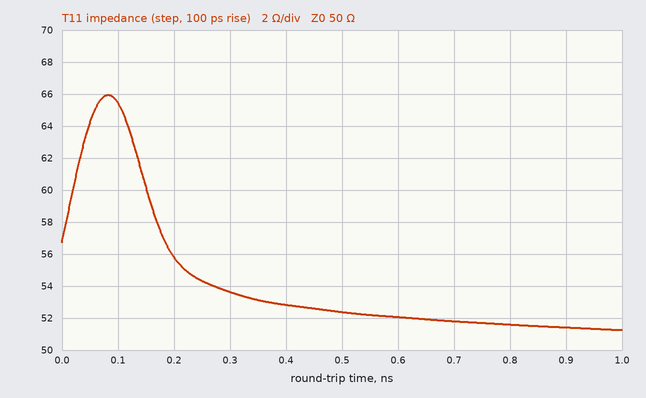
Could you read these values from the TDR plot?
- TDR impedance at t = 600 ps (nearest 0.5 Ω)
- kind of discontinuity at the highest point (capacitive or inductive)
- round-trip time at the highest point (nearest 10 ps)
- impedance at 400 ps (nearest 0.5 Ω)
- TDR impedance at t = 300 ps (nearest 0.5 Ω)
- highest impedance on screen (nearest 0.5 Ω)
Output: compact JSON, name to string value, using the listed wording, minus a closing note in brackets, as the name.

{"TDR impedance at t = 600 ps": "52.0 Ω", "kind of discontinuity at the highest point": "inductive", "round-trip time at the highest point": "80 ps", "impedance at 400 ps": "53.0 Ω", "TDR impedance at t = 300 ps": "53.5 Ω", "highest impedance on screen": "66.0 Ω"}
